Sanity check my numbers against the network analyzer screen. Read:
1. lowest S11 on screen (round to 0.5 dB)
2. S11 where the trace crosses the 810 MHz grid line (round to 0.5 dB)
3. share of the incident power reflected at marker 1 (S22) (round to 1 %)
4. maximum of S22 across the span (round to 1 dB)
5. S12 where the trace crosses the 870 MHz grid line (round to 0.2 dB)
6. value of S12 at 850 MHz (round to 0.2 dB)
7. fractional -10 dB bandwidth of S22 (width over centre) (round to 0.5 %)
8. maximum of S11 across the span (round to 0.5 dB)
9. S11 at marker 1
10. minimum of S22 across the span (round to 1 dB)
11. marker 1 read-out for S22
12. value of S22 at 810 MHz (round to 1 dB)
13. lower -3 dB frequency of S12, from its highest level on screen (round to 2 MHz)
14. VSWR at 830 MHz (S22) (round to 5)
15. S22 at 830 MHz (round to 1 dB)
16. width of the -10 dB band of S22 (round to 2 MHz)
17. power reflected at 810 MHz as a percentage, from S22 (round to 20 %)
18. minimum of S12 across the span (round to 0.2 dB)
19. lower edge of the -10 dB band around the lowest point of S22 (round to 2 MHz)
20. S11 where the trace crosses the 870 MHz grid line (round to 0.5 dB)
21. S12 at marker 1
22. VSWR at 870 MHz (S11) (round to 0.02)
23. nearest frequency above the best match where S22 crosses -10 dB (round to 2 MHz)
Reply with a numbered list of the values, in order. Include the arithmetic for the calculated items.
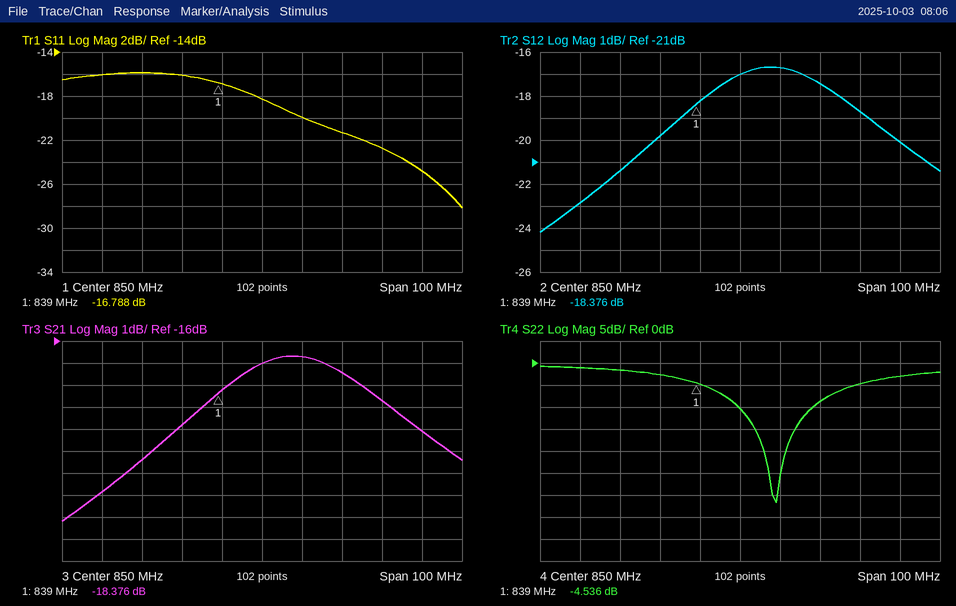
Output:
1. -28.0 dB
2. -16.0 dB
3. 10^(-4.536/10) ≈ 35 %
4. -1 dB
5. -17.4 dB
6. -17.0 dB
7. 18 MHz / 859 MHz ≈ 2.10 %, so 2.0 % to the nearest 0.5 %
8. -16.0 dB
9. -16.788 dB
10. -32 dB
11. -4.536 dB
12. -1 dB
13. 830 MHz
14. |Γ| = 10^(-3/20) = 0.7079; VSWR = (1 + 0.7079)/(1 − 0.7079) ≈ 5.85, so 5 to the nearest 5
15. -3 dB
16. 868 MHz − 850 MHz = 18 MHz
17. 10^(-1/10) ≈ 79.4 %, so 80 % to the nearest 20 %
18. -24.2 dB
19. 850 MHz
20. -21.5 dB
21. -18.376 dB
22. |Γ| = 10^(-21.5/20) = 0.0841; VSWR = (1 + 0.0841)/(1 − 0.0841) ≈ 1.18
23. 868 MHz
